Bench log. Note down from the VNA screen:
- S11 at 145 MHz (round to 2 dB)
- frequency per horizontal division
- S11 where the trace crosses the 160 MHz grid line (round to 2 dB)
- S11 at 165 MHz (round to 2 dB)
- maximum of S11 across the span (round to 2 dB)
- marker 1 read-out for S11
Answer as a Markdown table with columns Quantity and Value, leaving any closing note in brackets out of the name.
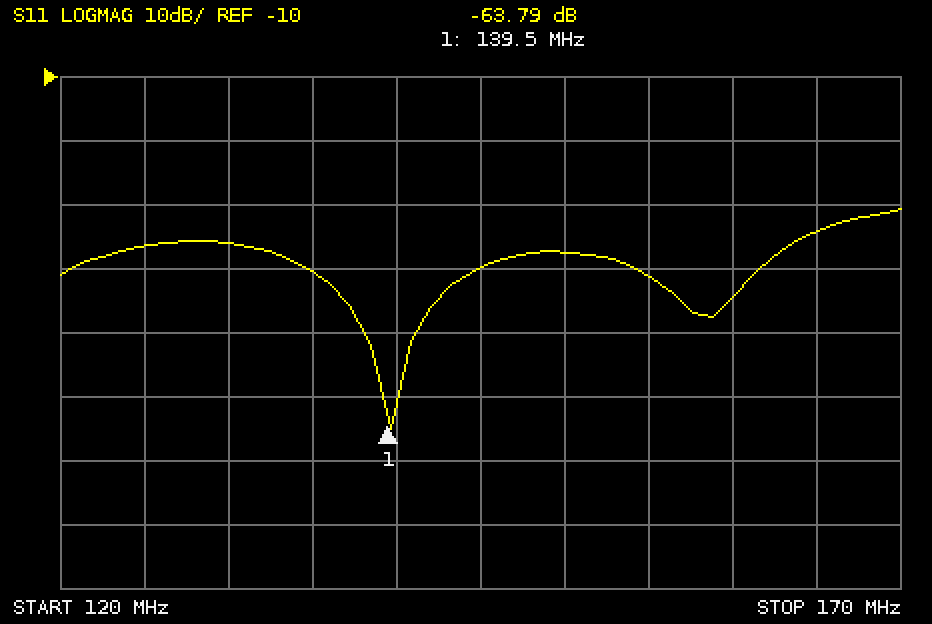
| Quantity | Value |
|---|---|
| S11 at 145 MHz | -40 dB |
| frequency per horizontal division | 5 MHz |
| S11 where the trace crosses the 160 MHz grid line | -44 dB |
| S11 at 165 MHz | -34 dB |
| maximum of S11 across the span | -30 dB |
| marker 1 read-out for S11 | -63.79 dB |
